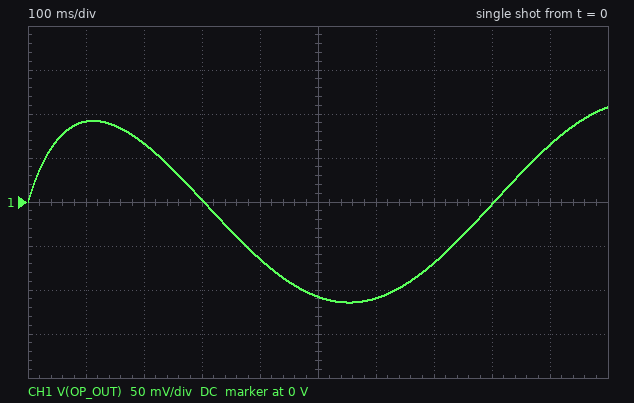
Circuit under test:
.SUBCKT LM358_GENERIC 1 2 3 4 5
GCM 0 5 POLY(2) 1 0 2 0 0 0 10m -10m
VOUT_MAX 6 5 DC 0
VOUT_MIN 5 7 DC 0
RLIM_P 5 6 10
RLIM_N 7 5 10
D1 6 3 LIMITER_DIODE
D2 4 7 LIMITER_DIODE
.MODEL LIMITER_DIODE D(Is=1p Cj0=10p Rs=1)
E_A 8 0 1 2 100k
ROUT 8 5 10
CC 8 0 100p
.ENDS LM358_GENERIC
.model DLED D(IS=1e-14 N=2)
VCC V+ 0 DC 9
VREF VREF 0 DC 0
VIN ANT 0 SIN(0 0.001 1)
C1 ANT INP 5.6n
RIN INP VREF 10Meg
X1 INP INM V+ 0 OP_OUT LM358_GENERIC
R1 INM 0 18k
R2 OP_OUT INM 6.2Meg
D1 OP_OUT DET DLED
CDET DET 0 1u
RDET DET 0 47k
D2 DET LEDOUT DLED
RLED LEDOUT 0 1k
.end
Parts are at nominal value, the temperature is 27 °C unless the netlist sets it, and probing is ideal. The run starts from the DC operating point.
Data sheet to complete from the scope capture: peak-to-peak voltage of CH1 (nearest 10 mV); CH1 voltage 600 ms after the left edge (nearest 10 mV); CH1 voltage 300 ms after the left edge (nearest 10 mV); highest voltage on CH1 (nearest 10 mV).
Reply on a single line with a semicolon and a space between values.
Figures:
220 mV; -110 mV; 0 V; 110 mV
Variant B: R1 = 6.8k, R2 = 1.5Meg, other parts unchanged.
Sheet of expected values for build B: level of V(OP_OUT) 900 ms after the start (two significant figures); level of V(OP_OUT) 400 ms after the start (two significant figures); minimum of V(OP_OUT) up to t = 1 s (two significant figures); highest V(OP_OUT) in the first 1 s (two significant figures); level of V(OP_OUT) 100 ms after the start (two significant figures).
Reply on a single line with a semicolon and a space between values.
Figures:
42 mV; -42 mV; -73 mV; 69 mV; 59 mV
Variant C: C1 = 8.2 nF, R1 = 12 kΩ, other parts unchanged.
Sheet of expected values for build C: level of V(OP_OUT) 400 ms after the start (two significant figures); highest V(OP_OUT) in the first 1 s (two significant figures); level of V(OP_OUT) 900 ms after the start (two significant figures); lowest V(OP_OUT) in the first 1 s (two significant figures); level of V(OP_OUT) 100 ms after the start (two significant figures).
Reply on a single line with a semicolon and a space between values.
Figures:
-110 mV; 210 mV; 110 mV; -240 mV; 170 mV
